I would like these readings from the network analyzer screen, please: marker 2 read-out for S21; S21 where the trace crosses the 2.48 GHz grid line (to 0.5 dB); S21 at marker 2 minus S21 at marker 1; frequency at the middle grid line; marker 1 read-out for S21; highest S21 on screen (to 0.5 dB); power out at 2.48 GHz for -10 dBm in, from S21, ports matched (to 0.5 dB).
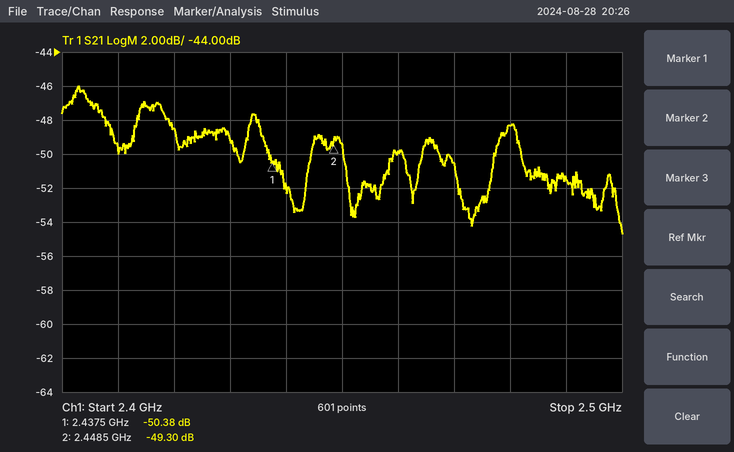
-49.30 dB
-48.5 dB
1.08 dB
2.45 GHz
-50.38 dB
-46.0 dB
-58.5 dBm
